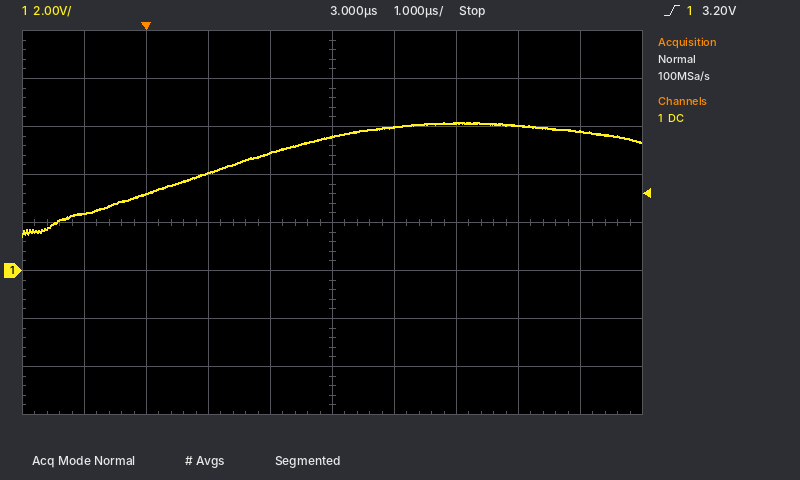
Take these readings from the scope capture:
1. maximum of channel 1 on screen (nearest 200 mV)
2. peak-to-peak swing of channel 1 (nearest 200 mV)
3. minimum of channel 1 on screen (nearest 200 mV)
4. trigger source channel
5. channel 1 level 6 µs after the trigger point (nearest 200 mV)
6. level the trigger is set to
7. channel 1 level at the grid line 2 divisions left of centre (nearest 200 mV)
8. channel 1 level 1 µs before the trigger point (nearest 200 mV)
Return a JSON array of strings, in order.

["6.2 V", "4.8 V", "1.4 V", "channel 1", "6.0 V", "3.20 V", "4.0 V", "2.4 V"]
